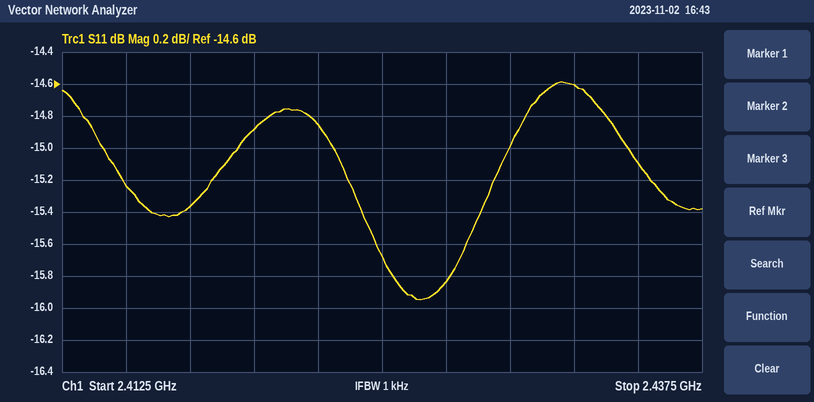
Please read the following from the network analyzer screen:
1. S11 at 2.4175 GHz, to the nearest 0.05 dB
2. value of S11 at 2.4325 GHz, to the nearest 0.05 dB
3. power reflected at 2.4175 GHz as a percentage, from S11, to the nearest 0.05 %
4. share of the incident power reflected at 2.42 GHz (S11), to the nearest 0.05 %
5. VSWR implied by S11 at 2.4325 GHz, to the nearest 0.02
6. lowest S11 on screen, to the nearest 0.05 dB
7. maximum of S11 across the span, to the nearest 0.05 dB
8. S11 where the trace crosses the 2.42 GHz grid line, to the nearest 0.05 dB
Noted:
-15.35 dB
-14.60 dB
2.90 %
3.25 %
1.46
-15.95 dB
-14.60 dB
-14.90 dB
